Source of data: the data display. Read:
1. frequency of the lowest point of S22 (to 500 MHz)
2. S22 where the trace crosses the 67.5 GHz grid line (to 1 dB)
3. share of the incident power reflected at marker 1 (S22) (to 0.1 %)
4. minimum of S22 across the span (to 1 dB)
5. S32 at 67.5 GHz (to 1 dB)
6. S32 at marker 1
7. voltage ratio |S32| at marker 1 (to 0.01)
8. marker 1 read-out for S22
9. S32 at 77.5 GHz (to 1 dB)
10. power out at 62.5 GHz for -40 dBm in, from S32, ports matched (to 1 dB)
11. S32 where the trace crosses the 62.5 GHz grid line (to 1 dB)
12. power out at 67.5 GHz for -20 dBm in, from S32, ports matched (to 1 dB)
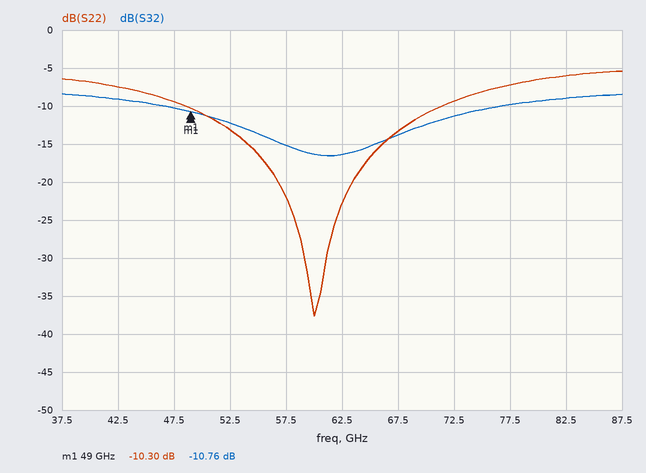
60.0 GHz
-13 dB
9.3 %
-38 dB
-14 dB
-10.76 dB
0.29
-10.30 dB
-10 dB
-56 dBm
-16 dB
-34 dBm
